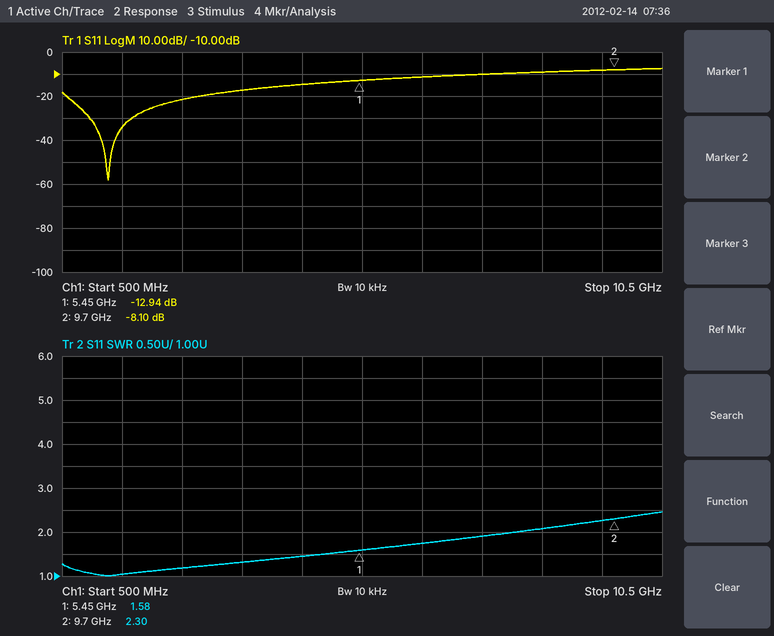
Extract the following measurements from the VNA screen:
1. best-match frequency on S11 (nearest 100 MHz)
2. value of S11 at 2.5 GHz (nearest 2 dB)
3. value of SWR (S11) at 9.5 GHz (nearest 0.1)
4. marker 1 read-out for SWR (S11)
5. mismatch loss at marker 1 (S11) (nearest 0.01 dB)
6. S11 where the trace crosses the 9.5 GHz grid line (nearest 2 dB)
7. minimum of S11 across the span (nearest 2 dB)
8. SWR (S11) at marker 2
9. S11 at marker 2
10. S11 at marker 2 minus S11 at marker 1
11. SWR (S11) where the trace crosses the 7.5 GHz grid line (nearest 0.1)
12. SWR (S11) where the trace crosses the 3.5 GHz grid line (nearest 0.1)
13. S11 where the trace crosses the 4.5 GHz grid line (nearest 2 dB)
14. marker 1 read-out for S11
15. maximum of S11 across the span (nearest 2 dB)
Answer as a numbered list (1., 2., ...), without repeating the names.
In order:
1. 1.3 GHz
2. -22 dB
3. 2.3
4. 1.58
5. 0.23 dB
6. -8 dB
7. -58 dB
8. 2.30
9. -8.10 dB
10. 4.84 dB
11. 1.9
12. 1.3
13. -14 dB
14. -12.94 dB
15. -8 dB
